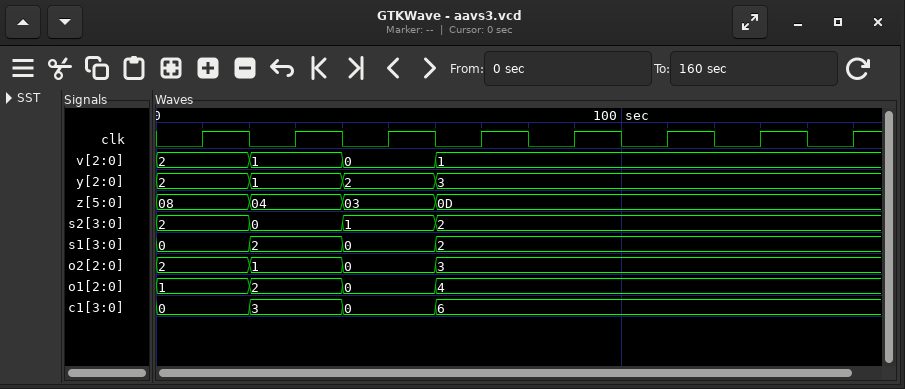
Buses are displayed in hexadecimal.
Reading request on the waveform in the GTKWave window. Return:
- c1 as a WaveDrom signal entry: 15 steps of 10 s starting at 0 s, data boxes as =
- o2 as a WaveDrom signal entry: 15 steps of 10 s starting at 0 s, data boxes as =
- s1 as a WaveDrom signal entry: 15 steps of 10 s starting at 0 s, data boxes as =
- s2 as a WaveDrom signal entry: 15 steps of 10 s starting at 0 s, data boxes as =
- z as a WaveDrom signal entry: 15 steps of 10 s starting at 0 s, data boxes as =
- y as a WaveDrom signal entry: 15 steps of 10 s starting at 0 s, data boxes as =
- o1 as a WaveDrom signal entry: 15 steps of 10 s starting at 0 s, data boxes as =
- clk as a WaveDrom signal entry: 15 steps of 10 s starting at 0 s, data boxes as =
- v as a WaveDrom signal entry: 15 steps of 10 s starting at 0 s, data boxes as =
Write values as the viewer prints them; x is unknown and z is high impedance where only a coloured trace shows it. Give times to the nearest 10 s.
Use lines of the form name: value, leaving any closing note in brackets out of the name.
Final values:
c1 as a WaveDrom signal entry: 15 steps of 10 s starting at 0 s, data boxes as =: {name: 'c1', wave: '=.=.=.=........', data: '0 3 0 6'}
o2 as a WaveDrom signal entry: 15 steps of 10 s starting at 0 s, data boxes as =: {name: 'o2', wave: '=.=.=.=........', data: '2 1 0 3'}
s1 as a WaveDrom signal entry: 15 steps of 10 s starting at 0 s, data boxes as =: {name: 's1', wave: '=.=.=.=........', data: '0 2 0 2'}
s2 as a WaveDrom signal entry: 15 steps of 10 s starting at 0 s, data boxes as =: {name: 's2', wave: '=.=.=.=........', data: '2 0 1 2'}
z as a WaveDrom signal entry: 15 steps of 10 s starting at 0 s, data boxes as =: {name: 'z', wave: '=.=.=.=........', data: '08 04 03 0D'}
y as a WaveDrom signal entry: 15 steps of 10 s starting at 0 s, data boxes as =: {name: 'y', wave: '=.=.=.=........', data: '2 1 2 3'}
o1 as a WaveDrom signal entry: 15 steps of 10 s starting at 0 s, data boxes as =: {name: 'o1', wave: '=.=.=.=........', data: '1 2 0 4'}
clk as a WaveDrom signal entry: 15 steps of 10 s starting at 0 s, data boxes as =: {name: 'clk', wave: '010101010101010'}
v as a WaveDrom signal entry: 15 steps of 10 s starting at 0 s, data boxes as =: {name: 'v', wave: '=.=.=.=........', data: '2 1 0 1'}
